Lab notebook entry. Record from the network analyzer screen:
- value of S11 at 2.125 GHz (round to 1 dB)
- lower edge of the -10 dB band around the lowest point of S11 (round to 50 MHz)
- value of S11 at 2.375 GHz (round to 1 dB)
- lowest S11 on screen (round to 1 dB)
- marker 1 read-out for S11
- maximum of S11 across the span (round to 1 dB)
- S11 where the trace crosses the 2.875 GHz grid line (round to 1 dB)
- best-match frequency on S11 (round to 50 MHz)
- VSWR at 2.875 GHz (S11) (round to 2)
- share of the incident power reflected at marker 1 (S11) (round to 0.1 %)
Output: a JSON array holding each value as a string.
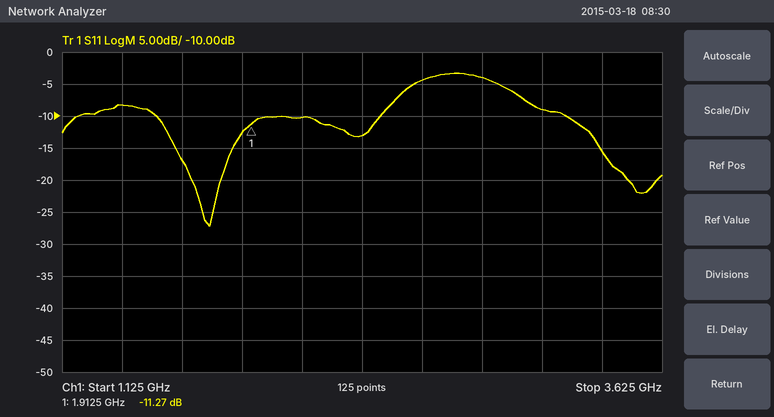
["-10 dB", "1.50 GHz", "-13 dB", "-27 dB", "-11.27 dB", "-3 dB", "-4 dB", "1.75 GHz", "4", "7.5 %"]
